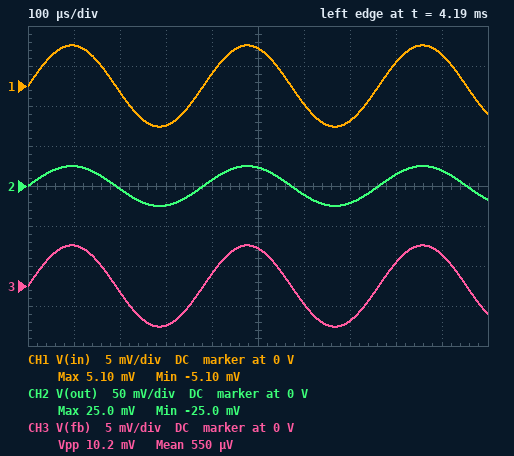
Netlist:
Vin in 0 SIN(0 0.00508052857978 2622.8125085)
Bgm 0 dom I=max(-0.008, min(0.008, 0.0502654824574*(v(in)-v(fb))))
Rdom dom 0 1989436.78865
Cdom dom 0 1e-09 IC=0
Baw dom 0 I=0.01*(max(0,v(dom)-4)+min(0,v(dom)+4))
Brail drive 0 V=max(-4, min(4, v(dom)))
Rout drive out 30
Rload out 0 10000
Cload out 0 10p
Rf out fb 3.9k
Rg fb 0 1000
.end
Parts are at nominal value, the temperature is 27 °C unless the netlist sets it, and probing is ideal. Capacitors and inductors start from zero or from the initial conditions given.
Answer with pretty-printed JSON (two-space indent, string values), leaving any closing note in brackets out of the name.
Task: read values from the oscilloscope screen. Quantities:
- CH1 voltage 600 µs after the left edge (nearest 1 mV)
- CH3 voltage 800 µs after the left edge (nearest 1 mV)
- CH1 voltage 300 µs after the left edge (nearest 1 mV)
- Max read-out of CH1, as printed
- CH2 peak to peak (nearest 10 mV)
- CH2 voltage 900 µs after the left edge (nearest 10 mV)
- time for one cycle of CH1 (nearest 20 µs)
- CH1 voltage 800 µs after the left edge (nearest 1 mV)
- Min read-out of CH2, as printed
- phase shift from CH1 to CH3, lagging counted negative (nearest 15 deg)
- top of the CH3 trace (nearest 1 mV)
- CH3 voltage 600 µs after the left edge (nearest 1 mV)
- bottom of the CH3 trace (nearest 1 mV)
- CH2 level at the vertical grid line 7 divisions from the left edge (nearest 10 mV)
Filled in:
{
  "CH1 voltage 600 µs after the left edge": "-2 mV",
  "CH3 voltage 800 µs after the left edge": "3 mV",
  "CH1 voltage 300 µs after the left edge": "-5 mV",
  "Max read-out of CH1, as printed": "5.10 mV",
  "CH2 peak to peak": "50 mV",
  "CH2 voltage 900 µs after the left edge": "20 mV",
  "time for one cycle of CH1": "380 µs",
  "CH1 voltage 800 µs after the left edge": "3 mV",
  "Min read-out of CH2, as printed": "-25.0 mV",
  "phase shift from CH1 to CH3, lagging counted negative": "0 deg",
  "top of the CH3 trace": "5 mV",
  "CH3 voltage 600 µs after the left edge": "-2 mV",
  "bottom of the CH3 trace": "-5 mV",
  "CH2 level at the vertical grid line 7 divisions from the left edge": "-20 mV"
}
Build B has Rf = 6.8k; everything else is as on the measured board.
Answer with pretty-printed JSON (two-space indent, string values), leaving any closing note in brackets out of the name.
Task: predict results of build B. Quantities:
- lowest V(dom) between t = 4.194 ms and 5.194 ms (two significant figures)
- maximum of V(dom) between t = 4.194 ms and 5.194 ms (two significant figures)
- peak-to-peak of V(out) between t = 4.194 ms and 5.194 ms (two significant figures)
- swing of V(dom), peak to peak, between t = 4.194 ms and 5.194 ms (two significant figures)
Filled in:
{
  "lowest V(dom) between t = 4.194 ms and 5.194 ms": "-40 mV",
  "maximum of V(dom) between t = 4.194 ms and 5.194 ms": "40 mV",
  "peak-to-peak of V(out) between t = 4.194 ms and 5.194 ms": "79 mV",
  "swing of V(dom), peak to peak, between t = 4.194 ms and 5.194 ms": "80 mV"
}
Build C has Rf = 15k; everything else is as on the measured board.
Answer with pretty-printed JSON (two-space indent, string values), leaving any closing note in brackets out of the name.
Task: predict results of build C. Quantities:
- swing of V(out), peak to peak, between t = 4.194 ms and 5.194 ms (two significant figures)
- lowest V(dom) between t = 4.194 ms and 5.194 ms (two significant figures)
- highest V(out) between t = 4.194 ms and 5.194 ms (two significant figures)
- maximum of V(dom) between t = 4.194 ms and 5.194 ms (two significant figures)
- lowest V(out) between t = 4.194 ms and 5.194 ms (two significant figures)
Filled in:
{
  "swing of V(out), peak to peak, between t = 4.194 ms and 5.194 ms": "160 mV",
  "lowest V(dom) between t = 4.194 ms and 5.194 ms": "-82 mV",
  "highest V(out) between t = 4.194 ms and 5.194 ms": "81 mV",
  "maximum of V(dom) between t = 4.194 ms and 5.194 ms": "82 mV",
  "lowest V(out) between t = 4.194 ms and 5.194 ms": "-81 mV"
}
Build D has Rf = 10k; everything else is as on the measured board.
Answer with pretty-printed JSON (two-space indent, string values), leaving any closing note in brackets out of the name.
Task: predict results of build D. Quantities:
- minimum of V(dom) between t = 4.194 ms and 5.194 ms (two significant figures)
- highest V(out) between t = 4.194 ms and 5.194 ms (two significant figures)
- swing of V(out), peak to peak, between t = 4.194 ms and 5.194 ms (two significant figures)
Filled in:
{
  "minimum of V(dom) between t = 4.194 ms and 5.194 ms": "-56 mV",
  "highest V(out) between t = 4.194 ms and 5.194 ms": "56 mV",
  "swing of V(out), peak to peak, between t = 4.194 ms and 5.194 ms": "110 mV"
}
